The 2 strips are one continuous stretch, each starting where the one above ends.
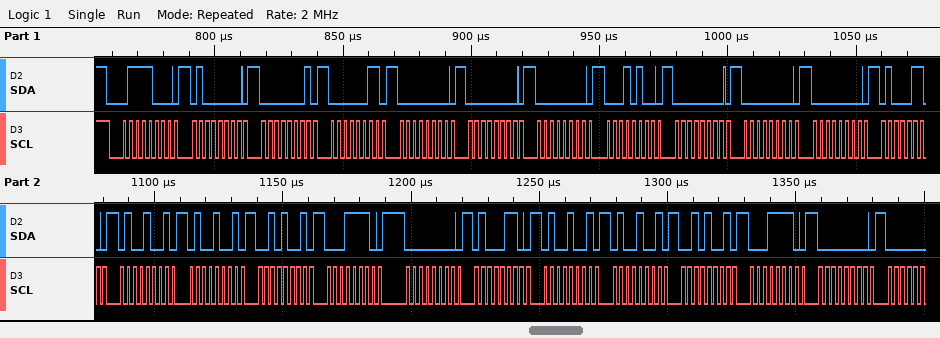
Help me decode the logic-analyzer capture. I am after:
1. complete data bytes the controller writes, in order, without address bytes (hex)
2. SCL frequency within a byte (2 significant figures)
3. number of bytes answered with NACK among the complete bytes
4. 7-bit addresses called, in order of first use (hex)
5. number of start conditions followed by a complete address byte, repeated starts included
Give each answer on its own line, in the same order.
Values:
40 01 03 00 00 00 14 00 00 00 46 49 49 29 1E 00 46 49 49 29 1E 00
400 kHz
0
0x3C
1
